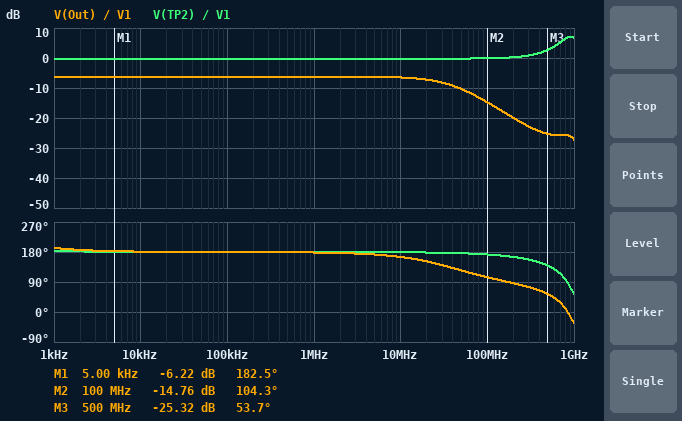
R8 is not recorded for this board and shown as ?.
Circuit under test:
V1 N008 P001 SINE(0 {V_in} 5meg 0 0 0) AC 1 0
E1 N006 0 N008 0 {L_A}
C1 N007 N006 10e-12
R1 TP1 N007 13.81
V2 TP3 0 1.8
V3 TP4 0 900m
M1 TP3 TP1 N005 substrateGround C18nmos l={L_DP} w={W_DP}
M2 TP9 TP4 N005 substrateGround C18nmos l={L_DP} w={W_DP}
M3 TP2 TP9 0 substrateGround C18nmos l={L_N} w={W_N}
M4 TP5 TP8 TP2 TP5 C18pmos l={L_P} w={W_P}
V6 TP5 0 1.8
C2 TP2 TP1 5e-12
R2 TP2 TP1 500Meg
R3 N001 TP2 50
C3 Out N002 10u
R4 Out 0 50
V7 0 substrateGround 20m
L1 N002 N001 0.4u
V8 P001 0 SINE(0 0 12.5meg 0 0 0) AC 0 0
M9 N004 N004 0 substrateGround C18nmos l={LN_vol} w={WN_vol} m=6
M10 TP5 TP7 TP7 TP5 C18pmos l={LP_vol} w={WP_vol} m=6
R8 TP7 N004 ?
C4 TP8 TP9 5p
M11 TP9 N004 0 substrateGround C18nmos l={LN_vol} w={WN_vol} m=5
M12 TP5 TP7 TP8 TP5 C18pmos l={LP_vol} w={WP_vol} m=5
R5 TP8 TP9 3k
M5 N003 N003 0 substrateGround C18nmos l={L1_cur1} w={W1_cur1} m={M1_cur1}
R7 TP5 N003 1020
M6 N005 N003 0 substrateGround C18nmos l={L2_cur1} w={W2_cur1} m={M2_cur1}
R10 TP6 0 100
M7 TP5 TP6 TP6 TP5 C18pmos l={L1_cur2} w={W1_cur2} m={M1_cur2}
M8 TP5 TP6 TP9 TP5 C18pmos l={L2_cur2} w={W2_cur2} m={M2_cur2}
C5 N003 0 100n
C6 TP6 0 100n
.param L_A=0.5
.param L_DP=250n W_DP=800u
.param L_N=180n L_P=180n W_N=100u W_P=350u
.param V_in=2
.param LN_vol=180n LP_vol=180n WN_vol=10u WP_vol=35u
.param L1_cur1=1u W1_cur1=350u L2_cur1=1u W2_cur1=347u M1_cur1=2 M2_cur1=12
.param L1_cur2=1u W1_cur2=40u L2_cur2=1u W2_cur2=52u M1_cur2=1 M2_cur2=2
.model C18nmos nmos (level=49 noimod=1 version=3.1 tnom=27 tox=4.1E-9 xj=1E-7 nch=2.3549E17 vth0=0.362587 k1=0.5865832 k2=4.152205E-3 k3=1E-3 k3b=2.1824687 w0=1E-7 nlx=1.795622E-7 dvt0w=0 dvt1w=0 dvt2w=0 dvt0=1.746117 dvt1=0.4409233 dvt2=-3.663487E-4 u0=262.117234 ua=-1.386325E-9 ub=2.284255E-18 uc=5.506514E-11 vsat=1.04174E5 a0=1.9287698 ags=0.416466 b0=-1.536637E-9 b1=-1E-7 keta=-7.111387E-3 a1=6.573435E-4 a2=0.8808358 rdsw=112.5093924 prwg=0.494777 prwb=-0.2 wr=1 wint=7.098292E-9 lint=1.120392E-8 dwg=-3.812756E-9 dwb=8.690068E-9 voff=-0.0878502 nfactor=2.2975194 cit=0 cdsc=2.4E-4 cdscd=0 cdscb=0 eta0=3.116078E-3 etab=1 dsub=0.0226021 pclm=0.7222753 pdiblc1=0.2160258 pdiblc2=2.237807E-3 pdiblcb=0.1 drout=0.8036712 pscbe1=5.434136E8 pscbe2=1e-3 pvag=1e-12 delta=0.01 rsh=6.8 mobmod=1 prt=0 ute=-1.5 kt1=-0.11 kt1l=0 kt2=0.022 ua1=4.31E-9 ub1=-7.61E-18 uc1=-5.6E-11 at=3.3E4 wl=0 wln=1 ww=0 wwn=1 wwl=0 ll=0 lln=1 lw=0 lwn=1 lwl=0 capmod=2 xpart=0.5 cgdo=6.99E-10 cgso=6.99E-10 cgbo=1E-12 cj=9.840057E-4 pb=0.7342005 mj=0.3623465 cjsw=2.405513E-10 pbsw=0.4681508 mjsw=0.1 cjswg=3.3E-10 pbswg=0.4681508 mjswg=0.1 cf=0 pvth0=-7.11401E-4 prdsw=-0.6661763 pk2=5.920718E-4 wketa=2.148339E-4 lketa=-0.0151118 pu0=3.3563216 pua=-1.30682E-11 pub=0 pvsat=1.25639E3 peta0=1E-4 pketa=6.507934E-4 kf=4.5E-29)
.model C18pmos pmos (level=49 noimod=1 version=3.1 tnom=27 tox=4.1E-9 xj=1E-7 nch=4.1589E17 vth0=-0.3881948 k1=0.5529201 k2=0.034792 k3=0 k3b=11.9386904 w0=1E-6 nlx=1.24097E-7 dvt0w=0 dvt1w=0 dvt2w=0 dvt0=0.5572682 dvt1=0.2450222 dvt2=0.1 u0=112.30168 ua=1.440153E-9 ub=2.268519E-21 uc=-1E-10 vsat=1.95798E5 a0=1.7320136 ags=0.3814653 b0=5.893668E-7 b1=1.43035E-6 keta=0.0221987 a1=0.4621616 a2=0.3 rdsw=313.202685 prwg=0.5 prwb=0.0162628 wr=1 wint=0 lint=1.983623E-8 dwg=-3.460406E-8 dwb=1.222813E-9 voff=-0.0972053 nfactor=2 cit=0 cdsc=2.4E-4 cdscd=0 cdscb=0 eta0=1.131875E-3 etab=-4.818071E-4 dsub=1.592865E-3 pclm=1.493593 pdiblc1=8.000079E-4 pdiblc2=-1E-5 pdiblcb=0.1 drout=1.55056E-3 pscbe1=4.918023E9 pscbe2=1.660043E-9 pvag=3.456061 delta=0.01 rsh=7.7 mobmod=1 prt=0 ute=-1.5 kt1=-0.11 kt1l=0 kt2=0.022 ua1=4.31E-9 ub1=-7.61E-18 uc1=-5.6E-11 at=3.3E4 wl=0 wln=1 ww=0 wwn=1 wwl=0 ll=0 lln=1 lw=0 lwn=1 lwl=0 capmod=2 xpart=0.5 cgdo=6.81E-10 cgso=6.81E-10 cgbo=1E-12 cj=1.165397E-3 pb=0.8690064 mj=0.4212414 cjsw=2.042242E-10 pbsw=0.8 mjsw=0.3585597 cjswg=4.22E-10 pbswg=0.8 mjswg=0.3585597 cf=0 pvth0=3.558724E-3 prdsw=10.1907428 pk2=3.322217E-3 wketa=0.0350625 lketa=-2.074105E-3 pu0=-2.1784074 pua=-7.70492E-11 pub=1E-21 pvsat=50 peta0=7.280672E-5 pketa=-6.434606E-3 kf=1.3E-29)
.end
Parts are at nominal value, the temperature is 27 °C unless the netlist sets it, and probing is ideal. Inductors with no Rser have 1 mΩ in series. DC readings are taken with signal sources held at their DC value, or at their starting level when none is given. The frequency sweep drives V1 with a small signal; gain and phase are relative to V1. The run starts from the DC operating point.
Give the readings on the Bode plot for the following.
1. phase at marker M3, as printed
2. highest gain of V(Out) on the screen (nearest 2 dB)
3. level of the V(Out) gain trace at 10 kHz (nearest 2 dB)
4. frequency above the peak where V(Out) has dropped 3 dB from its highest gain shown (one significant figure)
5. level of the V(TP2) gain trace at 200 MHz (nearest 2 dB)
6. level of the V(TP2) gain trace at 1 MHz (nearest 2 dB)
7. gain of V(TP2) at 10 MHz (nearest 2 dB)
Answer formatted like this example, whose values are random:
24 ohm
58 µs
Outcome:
53.7 deg
-6 dB
-6 dB
40 MHz
0 dB
0 dB
0 dB
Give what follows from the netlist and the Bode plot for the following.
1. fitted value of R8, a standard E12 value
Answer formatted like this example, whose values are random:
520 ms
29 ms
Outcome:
4.7 kΩ
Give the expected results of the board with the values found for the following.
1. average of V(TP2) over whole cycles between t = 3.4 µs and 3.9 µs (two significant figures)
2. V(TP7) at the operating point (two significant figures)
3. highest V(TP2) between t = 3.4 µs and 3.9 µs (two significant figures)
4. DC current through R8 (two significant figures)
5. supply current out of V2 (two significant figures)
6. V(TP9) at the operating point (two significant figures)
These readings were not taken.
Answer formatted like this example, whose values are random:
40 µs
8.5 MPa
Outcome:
880 mV
1.3 V
1.6 V
160 µA
3.7 mA
690 mV
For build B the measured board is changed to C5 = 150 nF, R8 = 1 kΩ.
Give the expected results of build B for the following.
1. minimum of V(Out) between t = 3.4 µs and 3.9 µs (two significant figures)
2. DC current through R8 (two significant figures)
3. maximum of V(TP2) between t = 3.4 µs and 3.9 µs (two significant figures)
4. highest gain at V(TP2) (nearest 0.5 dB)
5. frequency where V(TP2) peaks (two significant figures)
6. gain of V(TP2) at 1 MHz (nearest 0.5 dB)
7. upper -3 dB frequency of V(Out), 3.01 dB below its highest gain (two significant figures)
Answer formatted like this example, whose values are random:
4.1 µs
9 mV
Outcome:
-330 mV
610 µA
960 mV
2.5 dB
130 MHz
-59.5 dB
150 MHz
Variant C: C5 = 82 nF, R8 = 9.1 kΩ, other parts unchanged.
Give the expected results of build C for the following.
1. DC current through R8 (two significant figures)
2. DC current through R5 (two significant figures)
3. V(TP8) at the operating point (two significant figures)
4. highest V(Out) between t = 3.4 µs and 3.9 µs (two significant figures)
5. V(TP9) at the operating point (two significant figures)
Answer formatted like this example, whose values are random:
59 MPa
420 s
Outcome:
89 µA
80 µA
1.0 V
360 mV
780 mV
